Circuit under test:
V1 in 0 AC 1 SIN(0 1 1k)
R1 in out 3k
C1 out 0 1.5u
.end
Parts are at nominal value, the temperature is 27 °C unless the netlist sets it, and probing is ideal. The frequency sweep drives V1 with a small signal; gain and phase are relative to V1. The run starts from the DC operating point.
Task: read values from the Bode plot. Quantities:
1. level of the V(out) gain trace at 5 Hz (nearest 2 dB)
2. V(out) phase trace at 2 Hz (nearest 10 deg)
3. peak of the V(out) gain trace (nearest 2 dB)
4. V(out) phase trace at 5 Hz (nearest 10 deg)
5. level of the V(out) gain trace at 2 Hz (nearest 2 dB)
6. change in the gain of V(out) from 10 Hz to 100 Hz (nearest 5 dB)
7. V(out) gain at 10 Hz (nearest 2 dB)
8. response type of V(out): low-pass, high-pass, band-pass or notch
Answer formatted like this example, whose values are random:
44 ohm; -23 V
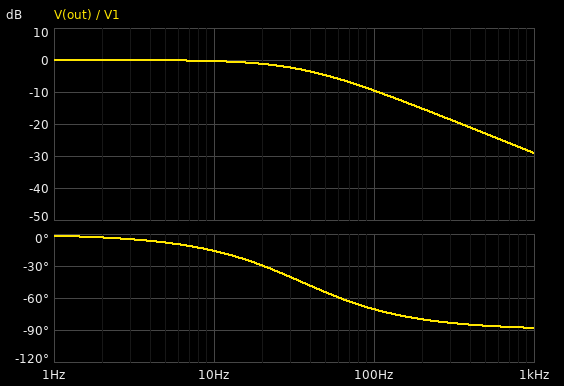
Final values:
0 dB; 0 deg; 0 dB; -10 deg; 0 dB; -10 dB; 0 dB; low-pass
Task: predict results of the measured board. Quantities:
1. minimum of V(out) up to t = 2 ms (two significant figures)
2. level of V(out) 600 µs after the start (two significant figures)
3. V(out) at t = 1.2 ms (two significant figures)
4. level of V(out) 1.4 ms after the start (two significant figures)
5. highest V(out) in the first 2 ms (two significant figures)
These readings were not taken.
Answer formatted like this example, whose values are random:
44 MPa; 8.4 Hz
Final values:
-13 mV; 59 mV; 17 mV; 55 mV; 67 mV
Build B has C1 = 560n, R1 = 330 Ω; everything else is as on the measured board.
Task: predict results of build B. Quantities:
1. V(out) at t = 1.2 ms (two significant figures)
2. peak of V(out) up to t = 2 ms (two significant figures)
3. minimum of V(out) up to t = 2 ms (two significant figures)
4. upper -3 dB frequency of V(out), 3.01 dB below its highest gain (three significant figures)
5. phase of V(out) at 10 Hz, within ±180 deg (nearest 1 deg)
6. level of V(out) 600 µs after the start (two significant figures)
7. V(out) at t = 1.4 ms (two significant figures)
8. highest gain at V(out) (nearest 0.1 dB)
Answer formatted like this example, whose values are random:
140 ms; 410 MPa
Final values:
250 mV; 720 mV; -650 mV; 861 Hz; -1 deg; 170 mV; 650 mV; 0 dB
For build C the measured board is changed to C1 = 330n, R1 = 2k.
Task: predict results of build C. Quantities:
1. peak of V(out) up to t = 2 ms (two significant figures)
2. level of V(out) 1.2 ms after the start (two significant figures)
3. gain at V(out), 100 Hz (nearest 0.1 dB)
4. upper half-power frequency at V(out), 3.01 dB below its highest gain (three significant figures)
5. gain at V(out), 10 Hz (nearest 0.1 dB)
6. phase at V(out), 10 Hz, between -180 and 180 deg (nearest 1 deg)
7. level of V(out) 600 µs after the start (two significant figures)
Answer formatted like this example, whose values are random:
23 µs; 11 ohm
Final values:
350 mV; 19 mV; -0.7 dB; 241 Hz; 0 dB; -2 deg; 240 mV
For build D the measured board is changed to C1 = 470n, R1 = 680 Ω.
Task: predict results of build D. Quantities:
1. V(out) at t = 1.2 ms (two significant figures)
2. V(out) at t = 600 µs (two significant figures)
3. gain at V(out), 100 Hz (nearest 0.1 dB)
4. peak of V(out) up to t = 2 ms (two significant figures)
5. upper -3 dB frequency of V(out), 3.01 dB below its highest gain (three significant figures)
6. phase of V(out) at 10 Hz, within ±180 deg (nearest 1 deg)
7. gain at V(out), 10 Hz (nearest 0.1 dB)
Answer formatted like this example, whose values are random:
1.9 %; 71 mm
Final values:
75 mV; 270 mV; -0.2 dB; 550 mV; 498 Hz; -1 deg; 0 dB
